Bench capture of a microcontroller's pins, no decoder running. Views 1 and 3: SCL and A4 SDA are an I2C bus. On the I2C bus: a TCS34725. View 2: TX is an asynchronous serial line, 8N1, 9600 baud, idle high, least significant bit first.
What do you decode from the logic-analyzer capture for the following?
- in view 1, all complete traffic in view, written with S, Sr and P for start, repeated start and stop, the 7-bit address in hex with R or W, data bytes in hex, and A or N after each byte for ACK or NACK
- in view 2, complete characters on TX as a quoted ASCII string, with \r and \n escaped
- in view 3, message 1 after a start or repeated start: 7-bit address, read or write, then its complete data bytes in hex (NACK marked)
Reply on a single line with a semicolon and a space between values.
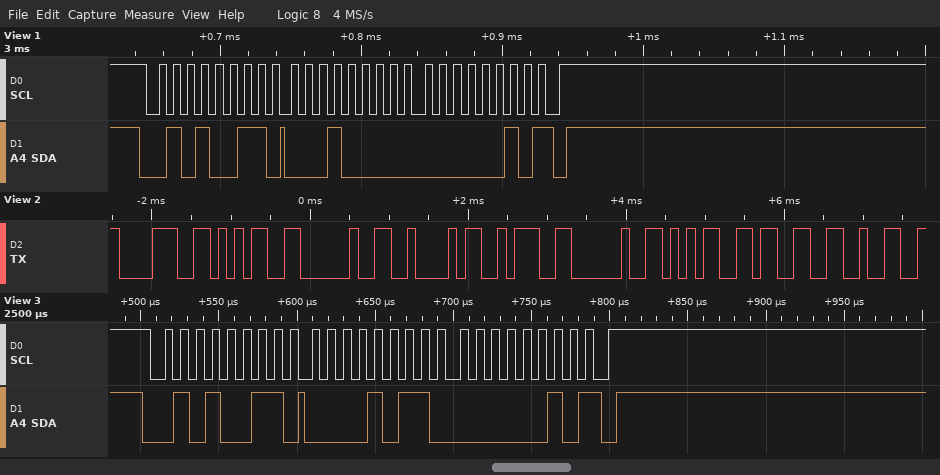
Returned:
S 29R A 10 A 02 N P; "85 B: 532"; 0x29 read: 0B 02 NACK
